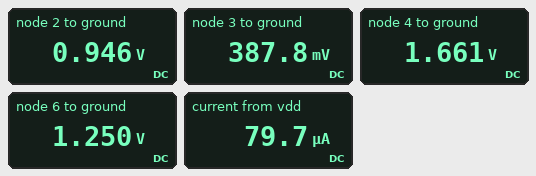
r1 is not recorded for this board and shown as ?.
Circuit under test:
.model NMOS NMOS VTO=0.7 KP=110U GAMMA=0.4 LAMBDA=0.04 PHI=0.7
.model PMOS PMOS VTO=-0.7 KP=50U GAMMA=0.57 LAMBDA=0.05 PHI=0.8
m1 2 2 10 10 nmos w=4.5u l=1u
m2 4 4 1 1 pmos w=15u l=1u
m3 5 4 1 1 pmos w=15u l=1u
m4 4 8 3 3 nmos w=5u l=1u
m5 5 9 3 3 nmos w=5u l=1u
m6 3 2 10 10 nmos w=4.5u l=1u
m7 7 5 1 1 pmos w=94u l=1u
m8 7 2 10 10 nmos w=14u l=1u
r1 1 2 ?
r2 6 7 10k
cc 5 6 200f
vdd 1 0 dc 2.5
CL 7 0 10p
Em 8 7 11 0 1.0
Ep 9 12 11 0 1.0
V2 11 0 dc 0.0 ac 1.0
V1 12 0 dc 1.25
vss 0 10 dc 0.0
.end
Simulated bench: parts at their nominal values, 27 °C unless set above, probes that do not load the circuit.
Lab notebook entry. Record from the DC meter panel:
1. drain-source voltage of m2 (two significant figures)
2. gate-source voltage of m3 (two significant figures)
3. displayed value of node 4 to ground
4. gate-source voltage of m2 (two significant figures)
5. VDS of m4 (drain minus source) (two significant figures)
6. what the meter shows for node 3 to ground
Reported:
-840 mV
-840 mV
1.661 V
-840 mV
1.3 V
387.8 mV
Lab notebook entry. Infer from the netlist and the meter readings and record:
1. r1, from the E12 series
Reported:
100 kΩ
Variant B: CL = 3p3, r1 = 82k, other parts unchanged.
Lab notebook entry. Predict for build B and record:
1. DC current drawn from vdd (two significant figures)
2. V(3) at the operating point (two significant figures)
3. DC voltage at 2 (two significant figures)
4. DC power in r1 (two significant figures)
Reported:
96 µA
370 mV
970 mV
29 µW
